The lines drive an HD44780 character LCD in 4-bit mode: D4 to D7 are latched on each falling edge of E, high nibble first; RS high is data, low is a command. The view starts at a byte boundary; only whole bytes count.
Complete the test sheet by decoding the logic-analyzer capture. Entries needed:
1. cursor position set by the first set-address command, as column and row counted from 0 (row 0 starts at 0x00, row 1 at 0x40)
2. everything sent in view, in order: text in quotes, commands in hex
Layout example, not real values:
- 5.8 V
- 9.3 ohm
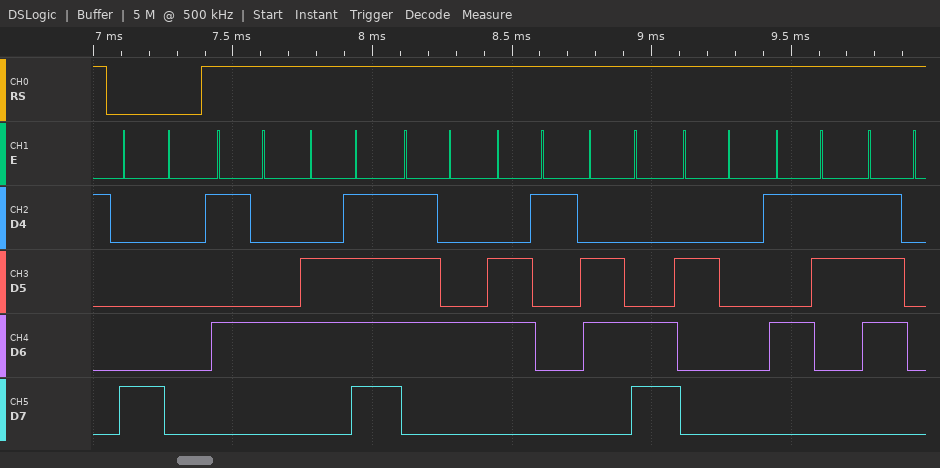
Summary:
- column 0, row 0
- 0x80 "Total Sp"
